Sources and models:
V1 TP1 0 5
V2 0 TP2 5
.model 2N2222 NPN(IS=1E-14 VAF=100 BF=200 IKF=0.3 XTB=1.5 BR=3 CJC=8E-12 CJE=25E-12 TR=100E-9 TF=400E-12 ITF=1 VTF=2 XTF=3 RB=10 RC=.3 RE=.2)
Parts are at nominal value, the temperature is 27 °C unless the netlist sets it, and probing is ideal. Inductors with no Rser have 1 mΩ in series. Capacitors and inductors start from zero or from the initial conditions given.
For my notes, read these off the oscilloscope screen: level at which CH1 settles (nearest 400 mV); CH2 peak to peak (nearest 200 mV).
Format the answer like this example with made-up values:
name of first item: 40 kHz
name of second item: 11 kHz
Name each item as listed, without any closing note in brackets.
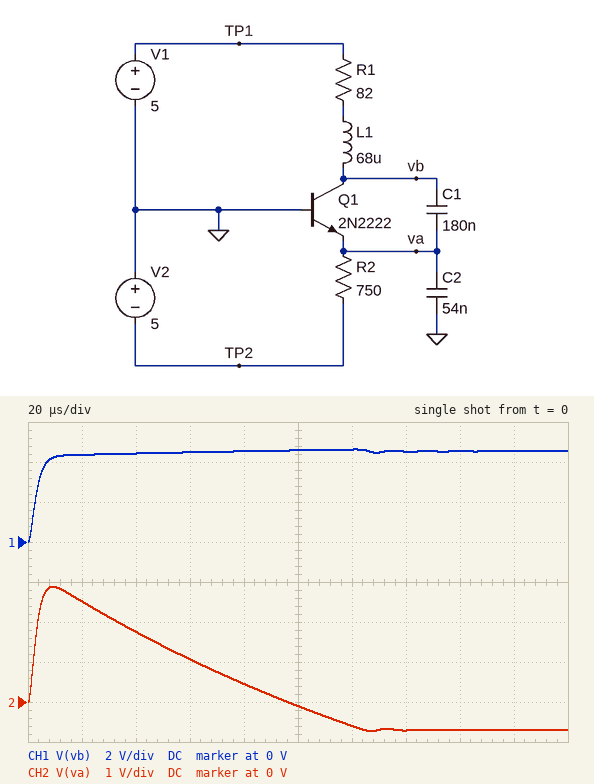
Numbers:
level at which CH1 settles: 4.4 V
CH2 peak to peak: 3.6 V
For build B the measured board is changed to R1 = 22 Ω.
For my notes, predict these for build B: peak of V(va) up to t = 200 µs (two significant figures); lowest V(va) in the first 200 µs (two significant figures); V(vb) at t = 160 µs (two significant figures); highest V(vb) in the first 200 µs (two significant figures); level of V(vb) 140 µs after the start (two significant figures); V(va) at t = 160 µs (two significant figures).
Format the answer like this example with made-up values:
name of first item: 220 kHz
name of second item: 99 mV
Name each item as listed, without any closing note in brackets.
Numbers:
peak of V(va) up to t = 200 µs: 4.9 V
lowest V(va) in the first 200 µs: -760 mV
V(vb) at t = 160 µs: 4.7 V
highest V(vb) in the first 200 µs: 6.7 V
level of V(vb) 140 µs after the start: 4.8 V
V(va) at t = 160 µs: -680 mV
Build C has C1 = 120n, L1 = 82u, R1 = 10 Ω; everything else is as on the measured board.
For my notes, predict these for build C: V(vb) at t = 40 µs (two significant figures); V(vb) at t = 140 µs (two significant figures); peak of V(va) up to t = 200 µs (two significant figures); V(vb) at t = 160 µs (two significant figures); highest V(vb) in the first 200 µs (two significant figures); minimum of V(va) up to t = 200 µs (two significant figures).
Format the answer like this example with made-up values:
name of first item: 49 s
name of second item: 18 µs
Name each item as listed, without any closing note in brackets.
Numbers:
V(vb) at t = 40 µs: 5.2 V
V(vb) at t = 140 µs: 5.0 V
peak of V(va) up to t = 200 µs: 5.4 V
V(vb) at t = 160 µs: 5.5 V
highest V(vb) in the first 200 µs: 8.3 V
minimum of V(va) up to t = 200 µs: -800 mV
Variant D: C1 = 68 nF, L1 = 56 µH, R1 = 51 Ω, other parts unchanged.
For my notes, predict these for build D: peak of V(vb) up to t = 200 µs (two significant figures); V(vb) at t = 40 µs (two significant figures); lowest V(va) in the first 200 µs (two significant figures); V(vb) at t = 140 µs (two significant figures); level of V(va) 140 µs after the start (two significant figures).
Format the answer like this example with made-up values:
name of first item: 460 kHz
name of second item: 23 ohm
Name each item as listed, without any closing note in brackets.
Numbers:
peak of V(vb) up to t = 200 µs: 5.2 V
V(vb) at t = 40 µs: 4.8 V
lowest V(va) in the first 200 µs: -750 mV
V(vb) at t = 140 µs: 4.4 V
level of V(va) 140 µs after the start: -730 mV
